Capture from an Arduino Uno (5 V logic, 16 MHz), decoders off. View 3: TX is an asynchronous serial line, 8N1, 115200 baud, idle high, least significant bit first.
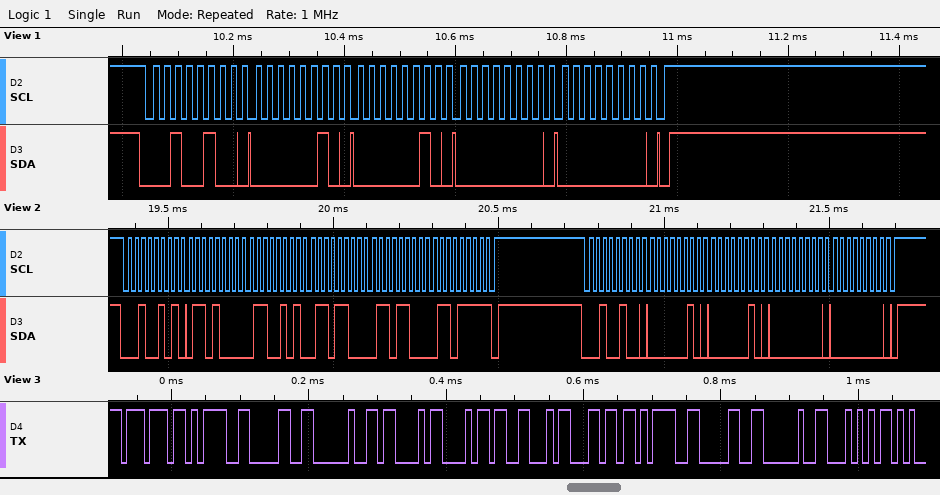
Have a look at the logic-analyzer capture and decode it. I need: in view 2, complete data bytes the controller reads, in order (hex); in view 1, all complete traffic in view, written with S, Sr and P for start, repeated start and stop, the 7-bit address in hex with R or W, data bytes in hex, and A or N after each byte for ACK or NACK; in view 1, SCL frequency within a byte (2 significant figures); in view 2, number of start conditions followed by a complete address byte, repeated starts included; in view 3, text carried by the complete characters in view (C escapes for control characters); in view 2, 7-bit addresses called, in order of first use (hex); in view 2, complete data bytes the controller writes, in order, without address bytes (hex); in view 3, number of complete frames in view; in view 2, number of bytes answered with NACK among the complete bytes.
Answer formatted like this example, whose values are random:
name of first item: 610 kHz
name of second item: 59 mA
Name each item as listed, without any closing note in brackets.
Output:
in view 2, complete data bytes the controller reads, in order: 68 65 6C 6C 6F
in view 1, all complete traffic in view, written with S, Sr and P for start, repeated start and stop, the 7-bit address in hex with R or W, data bytes in hex, and A or N after each byte for ACK or NACK: S 12W A 02 A 02 A 00 A 00 A P
in view 1, SCL frequency within a byte: 50 kHz
in view 2, number of start conditions followed by a complete address byte, repeated starts included: 2
in view 3, text carried by the complete characters in view: "w=0 ChFl=0 T"
in view 2, 7-bit addresses called, in order of first use: 0x12
in view 2, complete data bytes the controller writes, in order, without address bytes: 02 02 00 00
in view 3, number of complete frames in view: 12
in view 2, number of bytes answered with NACK among the complete bytes: 1
